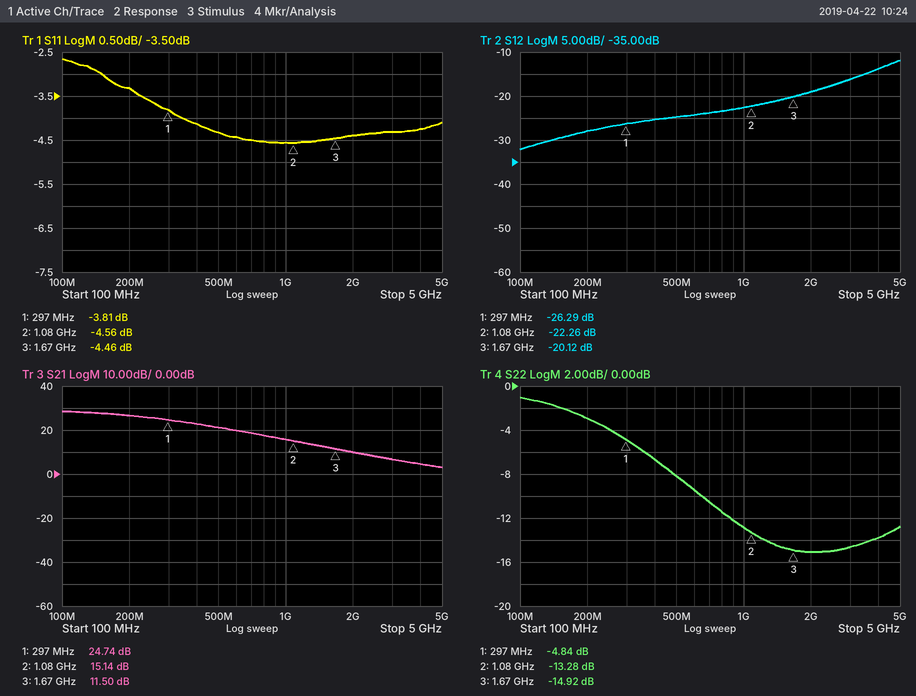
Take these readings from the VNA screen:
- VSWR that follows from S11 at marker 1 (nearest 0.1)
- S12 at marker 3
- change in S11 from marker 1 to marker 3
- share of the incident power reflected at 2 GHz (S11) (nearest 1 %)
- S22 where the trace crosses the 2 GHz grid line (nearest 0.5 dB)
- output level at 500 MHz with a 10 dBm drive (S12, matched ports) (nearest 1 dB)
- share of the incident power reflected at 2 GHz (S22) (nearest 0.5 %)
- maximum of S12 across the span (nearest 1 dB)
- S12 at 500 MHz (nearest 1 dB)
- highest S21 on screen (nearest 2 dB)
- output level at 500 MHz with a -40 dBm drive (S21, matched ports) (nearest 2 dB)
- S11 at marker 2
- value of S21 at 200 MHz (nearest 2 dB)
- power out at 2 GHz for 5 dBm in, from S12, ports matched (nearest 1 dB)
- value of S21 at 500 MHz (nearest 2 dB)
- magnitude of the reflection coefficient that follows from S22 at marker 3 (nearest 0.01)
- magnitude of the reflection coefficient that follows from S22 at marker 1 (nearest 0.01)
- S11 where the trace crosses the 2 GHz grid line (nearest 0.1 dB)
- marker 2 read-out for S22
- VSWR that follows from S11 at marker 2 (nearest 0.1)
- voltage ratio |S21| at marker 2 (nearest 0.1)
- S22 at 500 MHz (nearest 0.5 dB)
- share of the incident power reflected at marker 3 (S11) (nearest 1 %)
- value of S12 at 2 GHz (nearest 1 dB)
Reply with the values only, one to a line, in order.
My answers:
4.6
-20.12 dB
-0.65 dB
36 %
-15.0 dB
-15 dBm
3.0 %
-12 dB
-25 dB
28 dB
-18 dBm
-4.56 dB
26 dB
-14 dBm
22 dB
0.18
0.57
-4.4 dB
-13.28 dB
3.9
5.7
-8.0 dB
36 %
-19 dB
